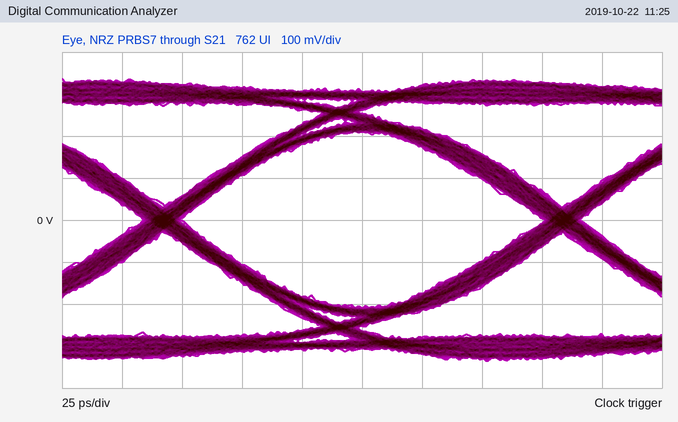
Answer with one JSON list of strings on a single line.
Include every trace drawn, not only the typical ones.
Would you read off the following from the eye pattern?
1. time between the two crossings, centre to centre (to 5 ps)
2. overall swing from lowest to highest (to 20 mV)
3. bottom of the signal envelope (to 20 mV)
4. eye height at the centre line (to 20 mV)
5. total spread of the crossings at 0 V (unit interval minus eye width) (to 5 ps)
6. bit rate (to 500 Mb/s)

["165 ps", "680 mV", "-340 mV", "420 mV", "15 ps", "6.0 Gb/s"]
